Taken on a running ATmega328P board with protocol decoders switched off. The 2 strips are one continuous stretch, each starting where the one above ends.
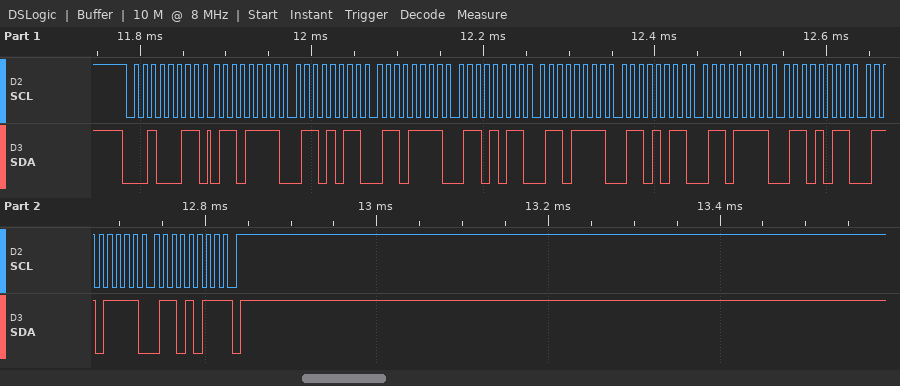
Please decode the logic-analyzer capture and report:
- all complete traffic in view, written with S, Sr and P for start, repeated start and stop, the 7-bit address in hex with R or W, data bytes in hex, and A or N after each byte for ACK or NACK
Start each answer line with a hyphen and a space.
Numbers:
- S 11R A 6F A 6B A 6F A 6B A 6F A 6B A 6F A 6B A 6F A 6B N P
